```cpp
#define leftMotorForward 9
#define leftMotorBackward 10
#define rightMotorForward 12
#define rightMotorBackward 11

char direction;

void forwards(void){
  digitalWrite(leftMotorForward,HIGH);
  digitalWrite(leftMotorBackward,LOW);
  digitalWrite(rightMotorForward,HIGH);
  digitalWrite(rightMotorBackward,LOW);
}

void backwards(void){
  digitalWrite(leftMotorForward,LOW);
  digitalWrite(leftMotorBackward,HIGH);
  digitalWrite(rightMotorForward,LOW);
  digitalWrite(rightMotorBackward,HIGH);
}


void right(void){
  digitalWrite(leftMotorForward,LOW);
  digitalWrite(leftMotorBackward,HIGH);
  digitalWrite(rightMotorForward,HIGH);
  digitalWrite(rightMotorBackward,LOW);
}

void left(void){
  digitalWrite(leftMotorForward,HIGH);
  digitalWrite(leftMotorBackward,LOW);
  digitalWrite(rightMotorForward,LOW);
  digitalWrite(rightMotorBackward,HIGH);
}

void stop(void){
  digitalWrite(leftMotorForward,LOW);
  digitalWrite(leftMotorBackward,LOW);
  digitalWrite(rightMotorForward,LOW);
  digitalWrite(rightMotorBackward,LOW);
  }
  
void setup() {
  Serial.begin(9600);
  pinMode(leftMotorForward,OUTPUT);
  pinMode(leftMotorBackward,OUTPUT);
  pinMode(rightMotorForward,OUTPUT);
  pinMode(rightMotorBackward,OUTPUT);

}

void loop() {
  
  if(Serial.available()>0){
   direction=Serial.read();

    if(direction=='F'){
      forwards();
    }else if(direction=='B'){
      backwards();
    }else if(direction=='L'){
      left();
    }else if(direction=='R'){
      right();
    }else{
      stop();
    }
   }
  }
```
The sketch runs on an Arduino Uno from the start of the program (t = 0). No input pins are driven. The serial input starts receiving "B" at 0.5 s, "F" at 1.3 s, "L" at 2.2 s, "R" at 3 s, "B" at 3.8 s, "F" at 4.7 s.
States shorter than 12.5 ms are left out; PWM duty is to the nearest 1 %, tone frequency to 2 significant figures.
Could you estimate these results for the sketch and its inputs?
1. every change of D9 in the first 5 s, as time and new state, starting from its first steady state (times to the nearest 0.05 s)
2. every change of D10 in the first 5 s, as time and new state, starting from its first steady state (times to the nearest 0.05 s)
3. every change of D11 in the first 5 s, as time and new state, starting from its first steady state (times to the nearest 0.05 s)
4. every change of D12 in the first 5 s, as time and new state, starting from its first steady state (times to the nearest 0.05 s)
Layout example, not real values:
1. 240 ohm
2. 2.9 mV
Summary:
1. 0 s low; 1.3 s high; 3 s low; 4.7 s high
2. 0 s low; 0.5 s high; 1.3 s low; 3 s high; 4.7 s low
3. 0 s low; 0.5 s high; 1.3 s low; 2.2 s high; 3 s low; 3.8 s high; 4.7 s low
4. 0 s low; 1.3 s high; 2.2 s low; 3 s high; 3.8 s low; 4.7 s high
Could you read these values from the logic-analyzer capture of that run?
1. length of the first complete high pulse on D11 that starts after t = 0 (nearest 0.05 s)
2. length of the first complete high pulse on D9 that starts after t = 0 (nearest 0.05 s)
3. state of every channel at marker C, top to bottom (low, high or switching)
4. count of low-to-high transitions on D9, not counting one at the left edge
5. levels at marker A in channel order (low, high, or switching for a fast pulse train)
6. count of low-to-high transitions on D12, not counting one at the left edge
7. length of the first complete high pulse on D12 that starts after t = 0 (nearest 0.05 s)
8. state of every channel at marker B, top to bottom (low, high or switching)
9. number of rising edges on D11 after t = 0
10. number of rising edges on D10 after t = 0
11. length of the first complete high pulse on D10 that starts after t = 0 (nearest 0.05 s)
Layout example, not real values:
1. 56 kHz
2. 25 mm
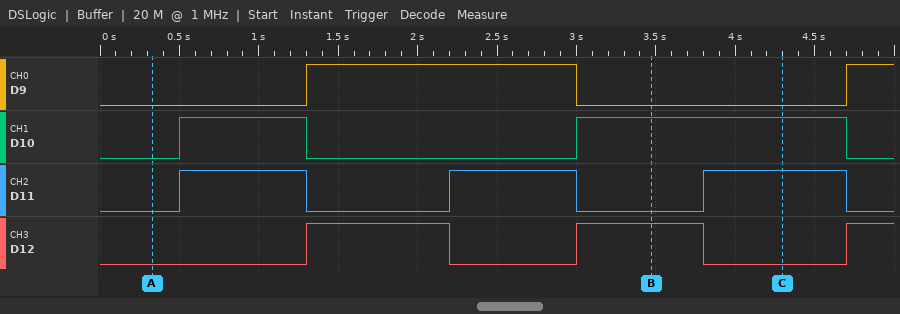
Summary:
1. 0.80 s
2. 1.70 s
3. D9 low, D10 high, D11 high, D12 low
4. 2
5. D9 low, D10 low, D11 low, D12 low
6. 3
7. 0.90 s
8. D9 low, D10 high, D11 low, D12 high
9. 3
10. 2
11. 0.80 s
